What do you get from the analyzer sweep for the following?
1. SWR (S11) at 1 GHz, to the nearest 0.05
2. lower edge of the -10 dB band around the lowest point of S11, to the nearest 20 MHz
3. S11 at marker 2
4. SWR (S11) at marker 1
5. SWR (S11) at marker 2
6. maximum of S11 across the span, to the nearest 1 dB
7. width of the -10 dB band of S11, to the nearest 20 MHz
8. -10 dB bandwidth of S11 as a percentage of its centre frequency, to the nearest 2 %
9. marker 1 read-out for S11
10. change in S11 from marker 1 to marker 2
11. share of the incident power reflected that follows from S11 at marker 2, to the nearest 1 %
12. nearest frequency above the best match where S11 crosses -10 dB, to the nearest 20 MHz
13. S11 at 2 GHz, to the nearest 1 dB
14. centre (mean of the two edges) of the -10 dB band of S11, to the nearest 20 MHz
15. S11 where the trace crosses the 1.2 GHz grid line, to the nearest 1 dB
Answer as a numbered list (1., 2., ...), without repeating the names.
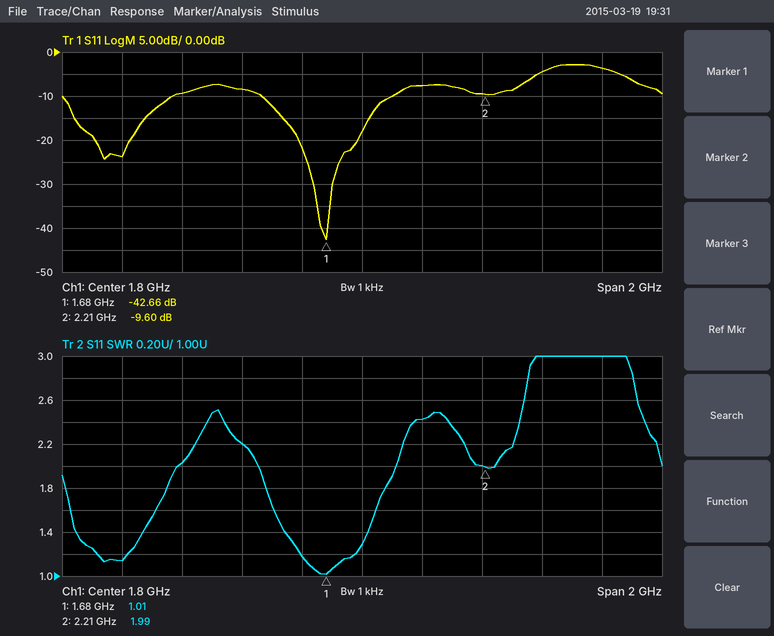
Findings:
1. 1.15
2. 1.46 GHz
3. -9.60 dB
4. 1.01
5. 1.99
6. -3 dB
7. 440 MHz
8. 26 %
9. -42.66 dB
10. 33.06 dB
11. 11 %
12. 1.90 GHz
13. -8 dB
14. 1.68 GHz
15. -9 dB
